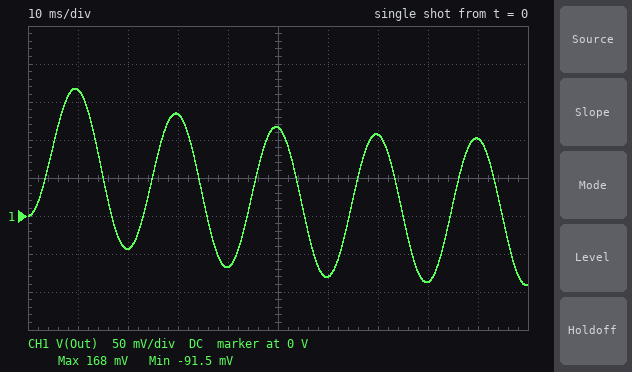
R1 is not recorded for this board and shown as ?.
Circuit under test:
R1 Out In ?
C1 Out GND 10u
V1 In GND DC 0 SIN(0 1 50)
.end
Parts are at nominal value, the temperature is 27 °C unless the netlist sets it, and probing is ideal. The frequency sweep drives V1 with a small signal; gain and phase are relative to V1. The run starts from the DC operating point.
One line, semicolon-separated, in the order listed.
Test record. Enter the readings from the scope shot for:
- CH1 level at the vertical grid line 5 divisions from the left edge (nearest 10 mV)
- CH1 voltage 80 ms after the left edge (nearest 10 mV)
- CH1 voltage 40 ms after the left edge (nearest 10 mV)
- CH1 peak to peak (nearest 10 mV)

120 mV; -90 mV; -70 mV; 260 mV
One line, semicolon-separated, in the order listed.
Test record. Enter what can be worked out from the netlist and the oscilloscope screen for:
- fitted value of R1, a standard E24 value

3.3 kΩ
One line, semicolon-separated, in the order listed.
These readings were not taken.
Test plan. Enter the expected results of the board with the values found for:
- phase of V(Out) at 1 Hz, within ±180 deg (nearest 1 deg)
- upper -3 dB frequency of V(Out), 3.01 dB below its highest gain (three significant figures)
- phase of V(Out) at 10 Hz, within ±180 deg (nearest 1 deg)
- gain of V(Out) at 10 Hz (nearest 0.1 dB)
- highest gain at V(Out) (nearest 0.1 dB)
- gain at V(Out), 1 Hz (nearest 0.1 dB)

-12 deg; 4.82 Hz; -64 deg; -7.2 dB; 0 dB; -0.2 dB
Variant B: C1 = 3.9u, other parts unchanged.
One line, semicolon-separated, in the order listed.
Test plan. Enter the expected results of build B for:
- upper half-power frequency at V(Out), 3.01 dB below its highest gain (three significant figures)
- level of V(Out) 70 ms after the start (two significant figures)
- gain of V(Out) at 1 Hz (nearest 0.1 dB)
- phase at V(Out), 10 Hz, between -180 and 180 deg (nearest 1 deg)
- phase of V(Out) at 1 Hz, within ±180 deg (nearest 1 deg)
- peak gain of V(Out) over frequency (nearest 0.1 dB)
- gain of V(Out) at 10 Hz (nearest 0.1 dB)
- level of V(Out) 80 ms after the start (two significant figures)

12.4 Hz; 230 mV; 0 dB; -39 deg; -5 deg; 0 dB; -2.2 dB; -230 mV
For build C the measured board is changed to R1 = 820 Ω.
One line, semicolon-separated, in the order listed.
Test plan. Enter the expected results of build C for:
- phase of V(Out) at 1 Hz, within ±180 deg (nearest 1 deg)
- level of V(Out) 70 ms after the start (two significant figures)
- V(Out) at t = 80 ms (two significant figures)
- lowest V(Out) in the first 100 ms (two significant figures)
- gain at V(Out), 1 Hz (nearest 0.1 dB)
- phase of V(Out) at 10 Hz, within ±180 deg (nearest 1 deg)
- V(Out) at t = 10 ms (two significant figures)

-3 deg; 340 mV; -340 mV; -360 mV; 0 dB; -27 deg; 440 mV
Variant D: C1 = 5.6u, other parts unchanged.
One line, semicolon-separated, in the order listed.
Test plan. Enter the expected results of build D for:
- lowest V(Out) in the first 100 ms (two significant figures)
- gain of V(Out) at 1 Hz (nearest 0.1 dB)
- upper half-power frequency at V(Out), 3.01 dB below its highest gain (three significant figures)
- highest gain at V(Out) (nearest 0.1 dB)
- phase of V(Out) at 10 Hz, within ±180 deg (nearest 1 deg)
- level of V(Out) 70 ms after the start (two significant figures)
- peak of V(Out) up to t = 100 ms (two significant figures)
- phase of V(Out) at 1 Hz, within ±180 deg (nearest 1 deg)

-170 mV; -0.1 dB; 8.61 Hz; 0 dB; -49 deg; 170 mV; 270 mV; -7 deg
